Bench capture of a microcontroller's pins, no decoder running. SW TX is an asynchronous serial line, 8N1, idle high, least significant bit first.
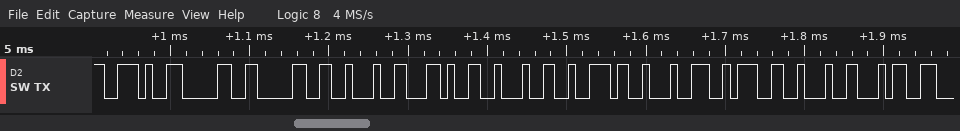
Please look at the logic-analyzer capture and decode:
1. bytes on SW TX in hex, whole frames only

0x2E 0x30 0x30 0x22 0x2C 0x22 0x72 0x22 0x3A 0x22 0x34
